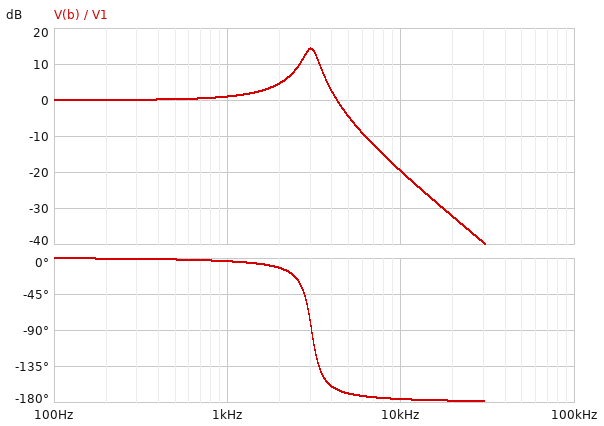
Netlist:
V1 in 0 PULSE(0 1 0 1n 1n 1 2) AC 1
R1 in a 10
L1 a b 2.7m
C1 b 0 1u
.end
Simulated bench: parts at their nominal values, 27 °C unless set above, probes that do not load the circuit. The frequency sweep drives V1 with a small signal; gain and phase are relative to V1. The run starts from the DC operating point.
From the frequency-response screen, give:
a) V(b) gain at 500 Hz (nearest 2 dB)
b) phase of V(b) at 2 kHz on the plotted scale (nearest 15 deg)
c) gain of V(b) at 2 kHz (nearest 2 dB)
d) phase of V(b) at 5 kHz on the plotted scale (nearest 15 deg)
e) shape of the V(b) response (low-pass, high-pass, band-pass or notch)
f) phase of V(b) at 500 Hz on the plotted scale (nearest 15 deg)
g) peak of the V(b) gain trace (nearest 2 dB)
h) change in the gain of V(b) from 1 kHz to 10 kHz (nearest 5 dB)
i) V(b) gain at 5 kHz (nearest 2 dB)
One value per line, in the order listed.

0 dB
-15 deg
4 dB
-165 deg
low-pass
0 deg
14 dB
-20 dB
-4 dB
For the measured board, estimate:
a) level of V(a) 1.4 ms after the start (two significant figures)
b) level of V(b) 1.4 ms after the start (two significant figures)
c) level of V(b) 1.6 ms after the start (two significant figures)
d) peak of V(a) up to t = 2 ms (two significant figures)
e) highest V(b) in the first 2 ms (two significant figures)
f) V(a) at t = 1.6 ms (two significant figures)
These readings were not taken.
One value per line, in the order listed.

990 mV
1.0 V
970 mV
1.1 V
1.7 V
1.0 V
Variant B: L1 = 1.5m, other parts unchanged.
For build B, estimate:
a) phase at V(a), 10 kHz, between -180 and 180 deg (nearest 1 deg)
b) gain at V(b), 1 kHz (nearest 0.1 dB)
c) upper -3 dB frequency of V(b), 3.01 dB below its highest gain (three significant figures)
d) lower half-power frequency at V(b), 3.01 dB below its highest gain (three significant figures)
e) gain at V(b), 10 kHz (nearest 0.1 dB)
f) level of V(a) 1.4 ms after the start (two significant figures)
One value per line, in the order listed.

7 deg
0.5 dB
4.54 kHz
3.46 kHz
-13.9 dB
1.0 V
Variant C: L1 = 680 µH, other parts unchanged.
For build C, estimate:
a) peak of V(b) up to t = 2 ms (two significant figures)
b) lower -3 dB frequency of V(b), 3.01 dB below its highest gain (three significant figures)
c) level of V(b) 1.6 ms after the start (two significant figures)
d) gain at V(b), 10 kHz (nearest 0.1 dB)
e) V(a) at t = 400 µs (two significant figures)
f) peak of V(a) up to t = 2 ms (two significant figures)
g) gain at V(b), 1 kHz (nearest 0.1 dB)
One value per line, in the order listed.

1.5 V
4.53 kHz
1.0 V
-5.1 dB
990 mV
1.2 V
0.2 dB
